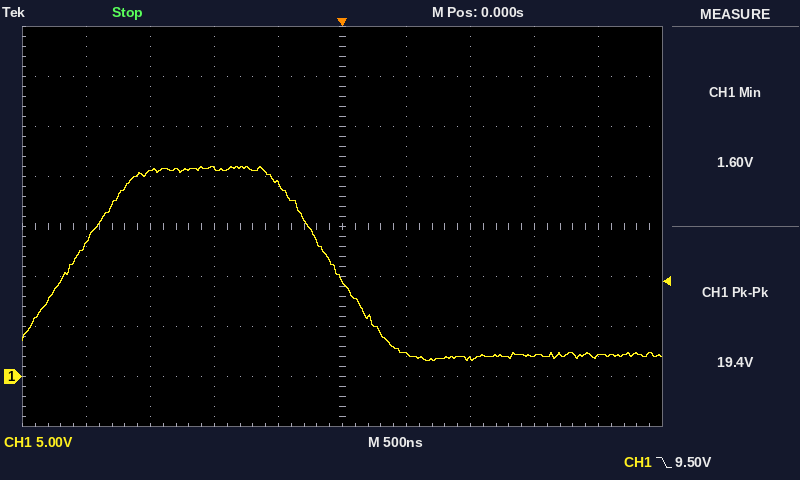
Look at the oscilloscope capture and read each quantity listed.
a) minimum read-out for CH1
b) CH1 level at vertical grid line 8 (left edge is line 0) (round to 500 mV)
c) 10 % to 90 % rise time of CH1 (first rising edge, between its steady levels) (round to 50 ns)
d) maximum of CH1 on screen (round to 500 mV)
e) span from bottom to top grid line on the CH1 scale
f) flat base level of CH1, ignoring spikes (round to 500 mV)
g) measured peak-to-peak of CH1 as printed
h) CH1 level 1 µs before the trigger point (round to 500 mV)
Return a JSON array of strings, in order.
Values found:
["1.60 V", "2.0 V", "800 ns", "21.0 V", "40 V", "2.0 V", "19.4 V", "21.0 V"]
